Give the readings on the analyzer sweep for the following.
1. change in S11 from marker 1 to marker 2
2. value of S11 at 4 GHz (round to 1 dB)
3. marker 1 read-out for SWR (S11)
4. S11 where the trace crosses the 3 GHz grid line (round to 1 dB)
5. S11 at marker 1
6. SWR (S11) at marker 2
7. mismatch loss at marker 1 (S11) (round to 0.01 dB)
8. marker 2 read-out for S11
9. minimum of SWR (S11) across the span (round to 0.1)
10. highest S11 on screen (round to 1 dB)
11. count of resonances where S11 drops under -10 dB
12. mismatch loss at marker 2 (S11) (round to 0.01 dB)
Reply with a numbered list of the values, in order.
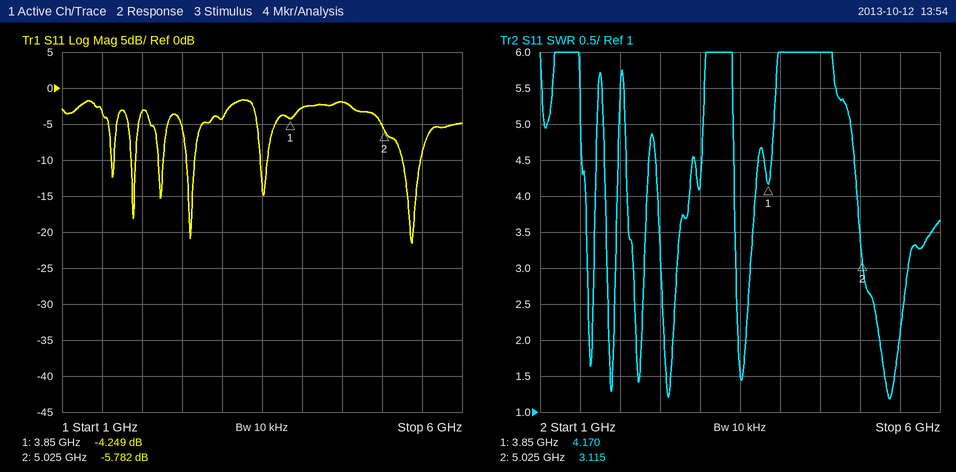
1. -1.533 dB
2. -3 dB
3. 4.170
4. -4 dB
5. -4.249 dB
6. 3.115
7. 2.05 dB
8. -5.782 dB
9. 1.2
10. -2 dB
11. 6
12. 1.33 dB
